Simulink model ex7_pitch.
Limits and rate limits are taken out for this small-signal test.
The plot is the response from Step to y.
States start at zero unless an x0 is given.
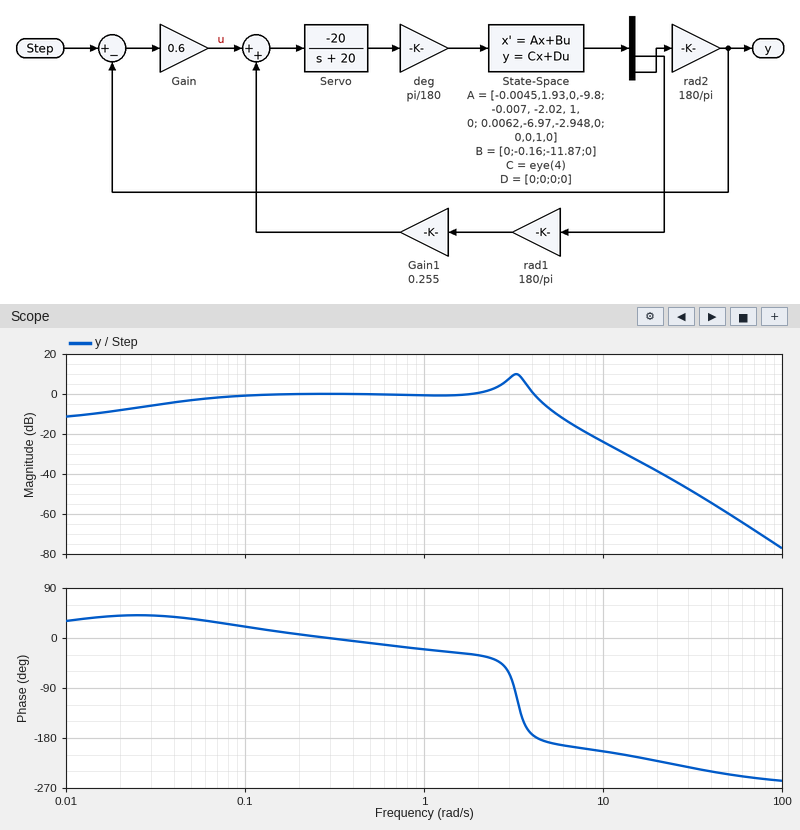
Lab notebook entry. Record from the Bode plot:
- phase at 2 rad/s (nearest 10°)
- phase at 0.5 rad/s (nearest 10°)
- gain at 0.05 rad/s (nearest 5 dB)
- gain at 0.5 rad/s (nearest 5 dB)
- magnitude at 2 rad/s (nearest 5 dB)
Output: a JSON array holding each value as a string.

["-30°", "-10°", "-5 dB", "0 dB", "0 dB"]
